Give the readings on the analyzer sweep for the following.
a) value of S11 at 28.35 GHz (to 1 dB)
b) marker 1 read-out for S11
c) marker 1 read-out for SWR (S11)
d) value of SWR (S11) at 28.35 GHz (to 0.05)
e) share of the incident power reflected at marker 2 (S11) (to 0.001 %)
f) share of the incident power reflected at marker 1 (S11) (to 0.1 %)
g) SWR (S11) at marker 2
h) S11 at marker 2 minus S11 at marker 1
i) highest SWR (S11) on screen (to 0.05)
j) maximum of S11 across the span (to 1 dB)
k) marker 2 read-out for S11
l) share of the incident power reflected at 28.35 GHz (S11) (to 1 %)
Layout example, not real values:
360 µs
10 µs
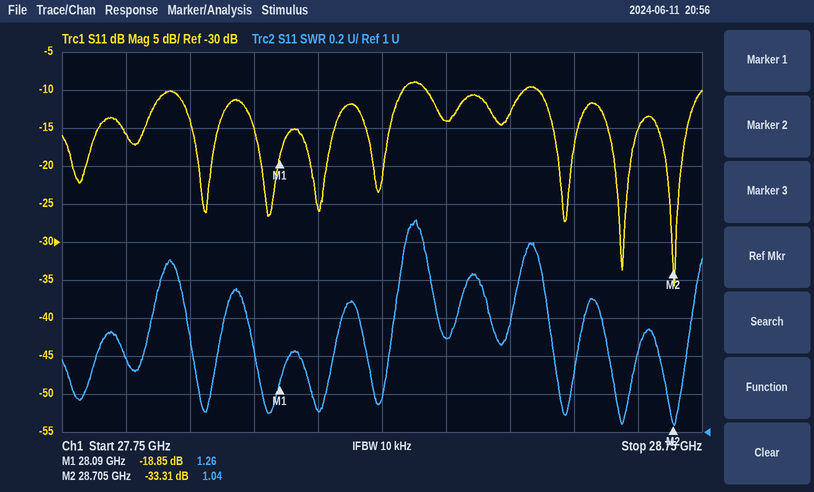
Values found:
-14 dB
-18.85 dB
1.26
1.50
0.047 %
1.3 %
1.04
-14.46 dB
2.10
-9 dB
-33.31 dB
4 %
